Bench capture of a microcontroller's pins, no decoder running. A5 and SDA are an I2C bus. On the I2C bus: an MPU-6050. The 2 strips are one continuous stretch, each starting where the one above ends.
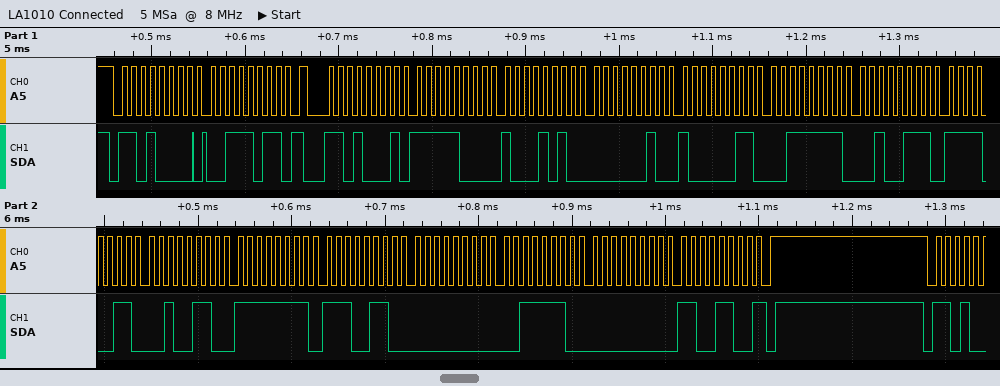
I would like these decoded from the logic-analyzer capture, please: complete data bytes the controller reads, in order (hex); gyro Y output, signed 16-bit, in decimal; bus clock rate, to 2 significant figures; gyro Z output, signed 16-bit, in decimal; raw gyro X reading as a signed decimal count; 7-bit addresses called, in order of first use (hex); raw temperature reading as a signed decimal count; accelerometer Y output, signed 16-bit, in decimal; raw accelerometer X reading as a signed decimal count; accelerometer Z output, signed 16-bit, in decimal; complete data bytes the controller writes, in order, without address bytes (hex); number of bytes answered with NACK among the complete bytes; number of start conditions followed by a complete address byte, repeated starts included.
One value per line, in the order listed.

F8 8A 02 83 3F 27 F3 26 FF E6 00 3E 00 CC
62
100 kHz
204
-26
0x68
-3290
643
-1910
16167
3B
1
2
